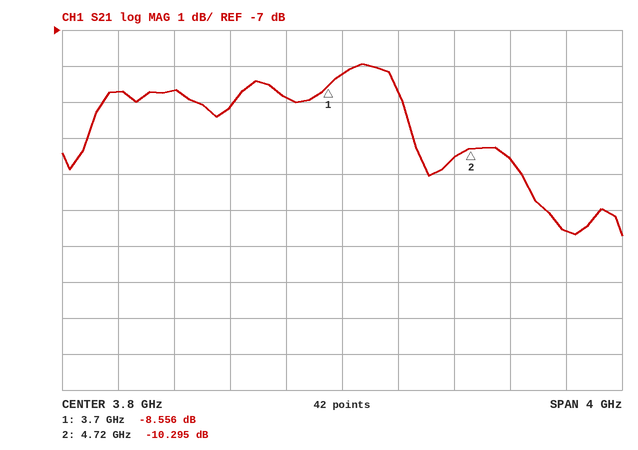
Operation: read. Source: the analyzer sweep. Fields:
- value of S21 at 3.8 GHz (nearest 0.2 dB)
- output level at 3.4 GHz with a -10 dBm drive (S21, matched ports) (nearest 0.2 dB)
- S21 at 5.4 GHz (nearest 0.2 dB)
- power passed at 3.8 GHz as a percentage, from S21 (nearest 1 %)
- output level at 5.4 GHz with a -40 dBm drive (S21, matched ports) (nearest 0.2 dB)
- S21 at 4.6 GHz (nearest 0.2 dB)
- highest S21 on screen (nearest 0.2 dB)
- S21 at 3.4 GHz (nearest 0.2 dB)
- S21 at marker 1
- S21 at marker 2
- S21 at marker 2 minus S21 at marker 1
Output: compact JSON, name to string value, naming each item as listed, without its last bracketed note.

{"value of S21 at 3.8 GHz": "-8.2 dB", "output level at 3.4 GHz with a -10 dBm drive (S21, matched ports)": "-18.8 dBm", "S21 at 5.4 GHz": "-12.6 dB", "power passed at 3.8 GHz as a percentage, from S21": "15 %", "output level at 5.4 GHz with a -40 dBm drive (S21, matched ports)": "-52.6 dBm", "S21 at 4.6 GHz": "-10.6 dB", "highest S21 on screen": "-8.0 dB", "S21 at 3.4 GHz": "-8.8 dB", "S21 at marker 1": "-8.556 dB", "S21 at marker 2": "-10.295 dB", "S21 at marker 2 minus S21 at marker 1": "-1.739 dB"}
